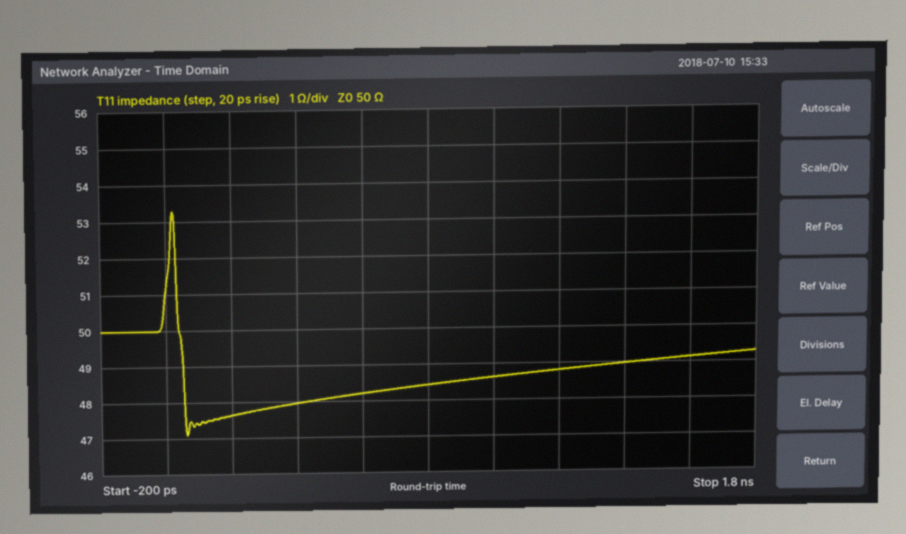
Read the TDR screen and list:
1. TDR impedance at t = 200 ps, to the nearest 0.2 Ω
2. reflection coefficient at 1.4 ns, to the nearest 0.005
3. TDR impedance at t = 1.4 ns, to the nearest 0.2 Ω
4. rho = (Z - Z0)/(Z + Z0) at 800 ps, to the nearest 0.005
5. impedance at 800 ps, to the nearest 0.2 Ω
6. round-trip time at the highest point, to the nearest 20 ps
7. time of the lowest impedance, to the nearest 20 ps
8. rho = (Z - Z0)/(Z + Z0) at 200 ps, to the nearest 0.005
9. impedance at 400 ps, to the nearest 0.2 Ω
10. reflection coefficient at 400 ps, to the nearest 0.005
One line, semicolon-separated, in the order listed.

47.6 Ω; -0.010; 49.0 Ω; -0.015; 48.4 Ω; 20 ps; 60 ps; -0.025; 48.0 Ω; -0.020
